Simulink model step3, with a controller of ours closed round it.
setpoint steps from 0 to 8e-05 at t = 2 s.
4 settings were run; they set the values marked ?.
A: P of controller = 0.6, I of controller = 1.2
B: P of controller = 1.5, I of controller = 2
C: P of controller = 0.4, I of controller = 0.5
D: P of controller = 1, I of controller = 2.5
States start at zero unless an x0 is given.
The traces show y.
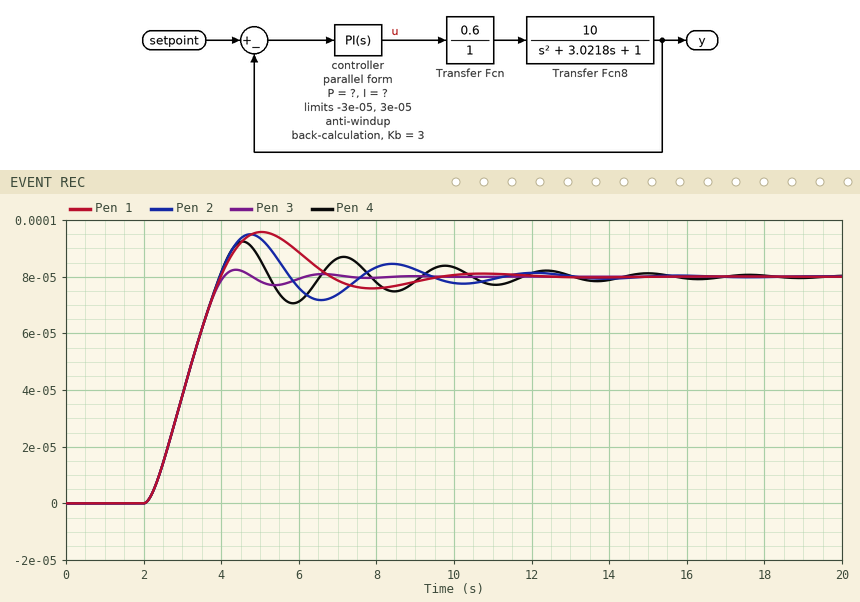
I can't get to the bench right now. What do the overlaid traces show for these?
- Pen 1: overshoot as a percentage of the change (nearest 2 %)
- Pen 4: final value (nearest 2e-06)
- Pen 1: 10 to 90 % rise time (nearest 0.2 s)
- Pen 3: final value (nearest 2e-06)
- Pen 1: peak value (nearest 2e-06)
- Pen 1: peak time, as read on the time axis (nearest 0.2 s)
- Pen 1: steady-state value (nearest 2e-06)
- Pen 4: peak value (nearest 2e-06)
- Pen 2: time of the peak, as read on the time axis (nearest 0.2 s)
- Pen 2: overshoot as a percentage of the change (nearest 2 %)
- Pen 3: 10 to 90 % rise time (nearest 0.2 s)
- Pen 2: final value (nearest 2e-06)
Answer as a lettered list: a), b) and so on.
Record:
a) 20 %
b) 0.000080
c) 1.4 s
d) 0.000080
e) 0.000096
f) 5.0 s
g) 0.000080
h) 0.000092
i) 4.8 s
j) 18 %
k) 1.4 s
l) 0.000080
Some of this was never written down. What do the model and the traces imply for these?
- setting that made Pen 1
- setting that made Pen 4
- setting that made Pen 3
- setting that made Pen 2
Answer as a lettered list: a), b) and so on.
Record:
a) C
b) D
c) B
d) A
